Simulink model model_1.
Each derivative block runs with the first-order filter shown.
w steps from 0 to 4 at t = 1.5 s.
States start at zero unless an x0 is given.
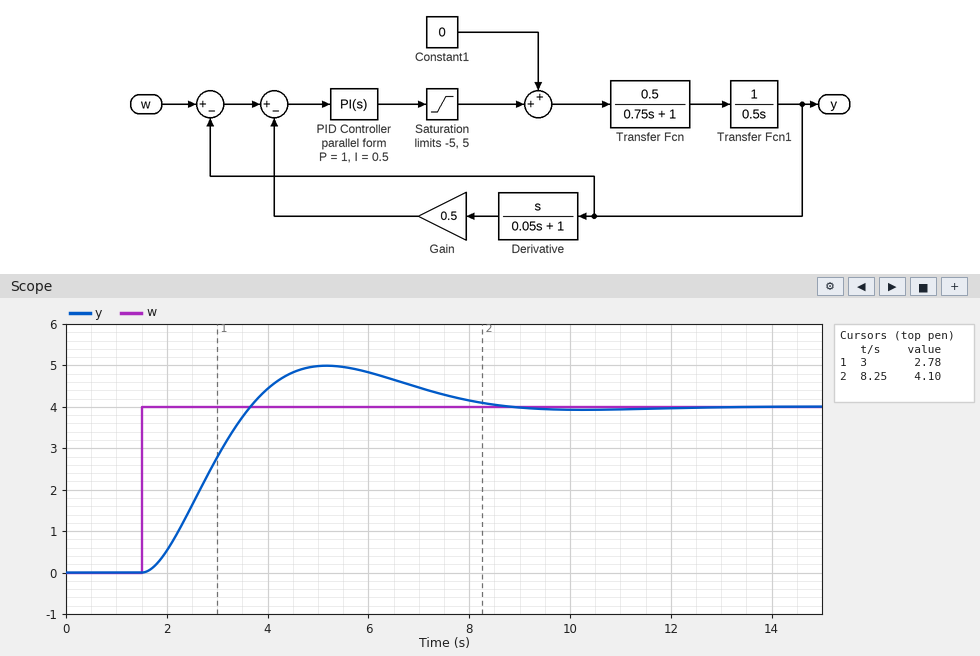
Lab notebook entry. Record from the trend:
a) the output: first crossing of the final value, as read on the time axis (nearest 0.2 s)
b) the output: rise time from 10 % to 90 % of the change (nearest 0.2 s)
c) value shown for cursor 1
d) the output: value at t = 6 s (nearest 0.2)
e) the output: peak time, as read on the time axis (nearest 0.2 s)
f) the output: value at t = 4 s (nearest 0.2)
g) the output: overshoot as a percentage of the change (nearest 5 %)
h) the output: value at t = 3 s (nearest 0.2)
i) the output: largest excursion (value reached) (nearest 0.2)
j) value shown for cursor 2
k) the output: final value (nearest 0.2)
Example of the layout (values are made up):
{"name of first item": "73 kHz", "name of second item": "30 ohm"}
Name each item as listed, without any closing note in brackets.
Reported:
{"the output: first crossing of the final value, as read on the time axis": "3.6 s", "the output: rise time from 10 % to 90 % of the change": "1.4 s", "value shown for cursor 1": "2.78", "the output: value at t = 6 s": "4.8", "the output: peak time, as read on the time axis": "5.2 s", "the output: value at t = 4 s": "4.4", "the output: overshoot as a percentage of the change": "25 %", "the output: value at t = 3 s": "2.8", "the output: largest excursion (value reached)": "5.0", "value shown for cursor 2": "4.10", "the output: final value": "4.0"}
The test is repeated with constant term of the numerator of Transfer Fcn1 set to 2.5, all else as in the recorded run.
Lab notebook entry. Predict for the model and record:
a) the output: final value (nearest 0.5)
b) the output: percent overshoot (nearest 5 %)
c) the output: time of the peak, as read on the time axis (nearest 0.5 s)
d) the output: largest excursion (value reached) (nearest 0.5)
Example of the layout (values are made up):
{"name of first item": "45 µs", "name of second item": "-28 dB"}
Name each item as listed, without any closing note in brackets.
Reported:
{"the output: final value": "4.0", "the output: percent overshoot": "10 %", "the output: time of the peak, as read on the time axis": "4.0 s", "the output: largest excursion (value reached)": "4.5"}
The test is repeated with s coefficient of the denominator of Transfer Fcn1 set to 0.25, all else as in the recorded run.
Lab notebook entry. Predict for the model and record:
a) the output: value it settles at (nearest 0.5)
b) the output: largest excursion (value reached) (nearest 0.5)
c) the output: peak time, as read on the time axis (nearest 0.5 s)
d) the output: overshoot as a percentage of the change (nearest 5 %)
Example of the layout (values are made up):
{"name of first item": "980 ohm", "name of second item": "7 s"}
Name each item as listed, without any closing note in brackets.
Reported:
{"the output: value it settles at": "4.0", "the output: largest excursion (value reached)": "4.5", "the output: peak time, as read on the time axis": "4.0 s", "the output: overshoot as a percentage of the change": "15 %"}
